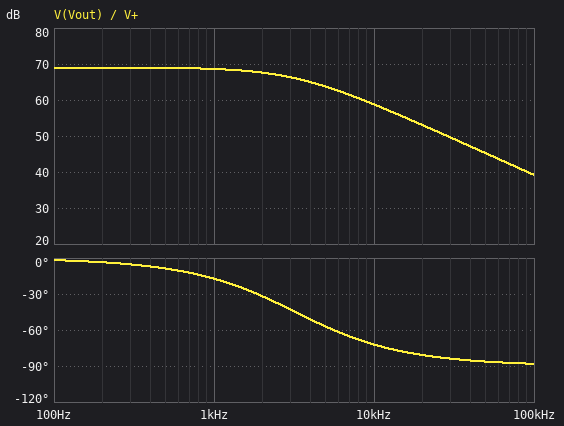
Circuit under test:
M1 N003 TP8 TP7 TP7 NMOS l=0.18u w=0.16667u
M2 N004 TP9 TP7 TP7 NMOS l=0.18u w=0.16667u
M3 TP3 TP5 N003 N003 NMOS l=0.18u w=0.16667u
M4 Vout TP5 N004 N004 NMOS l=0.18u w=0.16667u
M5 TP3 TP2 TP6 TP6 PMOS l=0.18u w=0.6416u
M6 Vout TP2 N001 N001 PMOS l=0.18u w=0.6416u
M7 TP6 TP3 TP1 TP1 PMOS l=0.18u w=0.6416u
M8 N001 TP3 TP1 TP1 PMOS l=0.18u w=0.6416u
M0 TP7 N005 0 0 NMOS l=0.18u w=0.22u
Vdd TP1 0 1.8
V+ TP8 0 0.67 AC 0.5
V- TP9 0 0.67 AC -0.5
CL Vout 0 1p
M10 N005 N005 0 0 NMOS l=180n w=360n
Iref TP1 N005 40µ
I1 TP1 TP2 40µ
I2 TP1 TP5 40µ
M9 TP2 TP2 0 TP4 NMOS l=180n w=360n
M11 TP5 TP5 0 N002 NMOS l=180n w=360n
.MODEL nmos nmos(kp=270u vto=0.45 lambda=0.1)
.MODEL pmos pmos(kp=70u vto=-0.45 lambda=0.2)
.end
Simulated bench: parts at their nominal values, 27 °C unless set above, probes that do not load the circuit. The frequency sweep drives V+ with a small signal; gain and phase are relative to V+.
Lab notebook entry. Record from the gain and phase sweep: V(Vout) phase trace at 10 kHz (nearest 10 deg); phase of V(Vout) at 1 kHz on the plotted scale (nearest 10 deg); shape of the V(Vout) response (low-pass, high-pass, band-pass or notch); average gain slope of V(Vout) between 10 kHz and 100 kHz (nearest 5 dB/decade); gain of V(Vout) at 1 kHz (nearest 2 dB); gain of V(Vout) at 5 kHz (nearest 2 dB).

-70 deg
-20 deg
low-pass
-20 dB/decade
68 dB
64 dB
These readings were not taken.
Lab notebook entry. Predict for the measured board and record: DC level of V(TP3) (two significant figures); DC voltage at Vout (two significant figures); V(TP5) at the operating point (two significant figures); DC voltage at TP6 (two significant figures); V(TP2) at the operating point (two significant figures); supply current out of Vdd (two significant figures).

1.2 V
1.2 V
820 mV
1.4 V
820 mV
130 µA
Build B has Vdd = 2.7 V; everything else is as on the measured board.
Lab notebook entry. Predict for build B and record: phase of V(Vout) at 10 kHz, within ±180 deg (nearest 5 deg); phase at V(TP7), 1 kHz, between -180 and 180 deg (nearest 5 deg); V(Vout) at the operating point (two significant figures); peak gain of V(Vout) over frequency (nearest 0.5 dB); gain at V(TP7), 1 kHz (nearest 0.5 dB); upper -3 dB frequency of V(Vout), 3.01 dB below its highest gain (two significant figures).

-5 deg
0 deg
2.1 V
40.5 dB
-19.0 dB
93 kHz
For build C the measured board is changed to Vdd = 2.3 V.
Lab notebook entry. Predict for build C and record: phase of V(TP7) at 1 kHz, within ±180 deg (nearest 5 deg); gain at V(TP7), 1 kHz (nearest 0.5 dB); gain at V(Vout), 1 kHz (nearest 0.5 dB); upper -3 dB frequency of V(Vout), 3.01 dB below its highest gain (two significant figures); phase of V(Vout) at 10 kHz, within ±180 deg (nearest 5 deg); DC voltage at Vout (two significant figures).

0 deg
-19.0 dB
40.5 dB
89 kHz
-5 deg
1.7 V
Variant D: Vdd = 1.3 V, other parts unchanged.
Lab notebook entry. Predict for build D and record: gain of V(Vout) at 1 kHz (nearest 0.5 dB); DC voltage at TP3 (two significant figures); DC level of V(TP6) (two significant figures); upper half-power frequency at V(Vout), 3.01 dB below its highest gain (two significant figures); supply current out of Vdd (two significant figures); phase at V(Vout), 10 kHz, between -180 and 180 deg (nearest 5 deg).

-44.5 dB
6.2 mV
1.3 V
4.2 MHz
120 µA
0 deg
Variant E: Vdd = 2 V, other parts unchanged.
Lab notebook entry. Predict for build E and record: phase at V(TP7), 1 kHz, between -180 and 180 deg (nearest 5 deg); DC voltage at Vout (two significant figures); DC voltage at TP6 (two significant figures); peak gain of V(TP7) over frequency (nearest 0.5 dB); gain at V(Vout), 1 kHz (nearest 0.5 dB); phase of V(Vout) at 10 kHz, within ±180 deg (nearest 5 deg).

0 deg
1.4 V
1.5 V
-19.0 dB
44.0 dB
-10 deg
